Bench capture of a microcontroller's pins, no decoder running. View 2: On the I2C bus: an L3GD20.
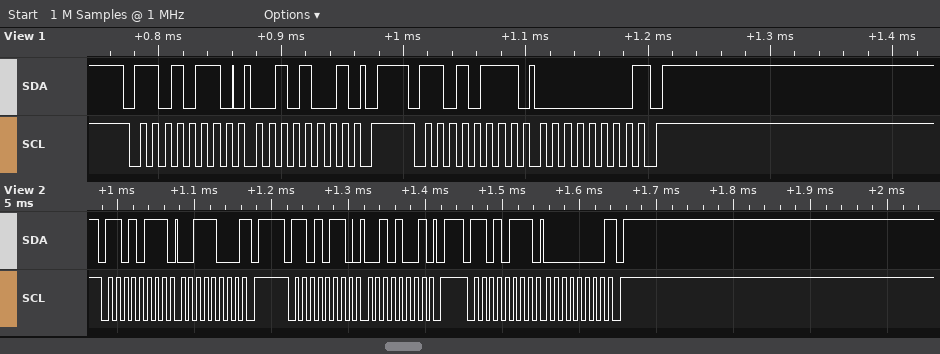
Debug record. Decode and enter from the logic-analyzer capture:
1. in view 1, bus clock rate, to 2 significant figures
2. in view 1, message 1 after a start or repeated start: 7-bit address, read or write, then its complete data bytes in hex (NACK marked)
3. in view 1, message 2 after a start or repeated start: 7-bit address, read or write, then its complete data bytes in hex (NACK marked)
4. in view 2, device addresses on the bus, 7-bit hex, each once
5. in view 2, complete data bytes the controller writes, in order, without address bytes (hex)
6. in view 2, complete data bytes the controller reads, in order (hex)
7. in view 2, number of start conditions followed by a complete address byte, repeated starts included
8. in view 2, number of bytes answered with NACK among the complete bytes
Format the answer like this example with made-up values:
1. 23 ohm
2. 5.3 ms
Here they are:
1. 100 kHz
2. 0x6B write: 29
3. 0x6B read: 00 NACK
4. 0x6B
5. 29
6. 38 00
7. 3
8. 2
